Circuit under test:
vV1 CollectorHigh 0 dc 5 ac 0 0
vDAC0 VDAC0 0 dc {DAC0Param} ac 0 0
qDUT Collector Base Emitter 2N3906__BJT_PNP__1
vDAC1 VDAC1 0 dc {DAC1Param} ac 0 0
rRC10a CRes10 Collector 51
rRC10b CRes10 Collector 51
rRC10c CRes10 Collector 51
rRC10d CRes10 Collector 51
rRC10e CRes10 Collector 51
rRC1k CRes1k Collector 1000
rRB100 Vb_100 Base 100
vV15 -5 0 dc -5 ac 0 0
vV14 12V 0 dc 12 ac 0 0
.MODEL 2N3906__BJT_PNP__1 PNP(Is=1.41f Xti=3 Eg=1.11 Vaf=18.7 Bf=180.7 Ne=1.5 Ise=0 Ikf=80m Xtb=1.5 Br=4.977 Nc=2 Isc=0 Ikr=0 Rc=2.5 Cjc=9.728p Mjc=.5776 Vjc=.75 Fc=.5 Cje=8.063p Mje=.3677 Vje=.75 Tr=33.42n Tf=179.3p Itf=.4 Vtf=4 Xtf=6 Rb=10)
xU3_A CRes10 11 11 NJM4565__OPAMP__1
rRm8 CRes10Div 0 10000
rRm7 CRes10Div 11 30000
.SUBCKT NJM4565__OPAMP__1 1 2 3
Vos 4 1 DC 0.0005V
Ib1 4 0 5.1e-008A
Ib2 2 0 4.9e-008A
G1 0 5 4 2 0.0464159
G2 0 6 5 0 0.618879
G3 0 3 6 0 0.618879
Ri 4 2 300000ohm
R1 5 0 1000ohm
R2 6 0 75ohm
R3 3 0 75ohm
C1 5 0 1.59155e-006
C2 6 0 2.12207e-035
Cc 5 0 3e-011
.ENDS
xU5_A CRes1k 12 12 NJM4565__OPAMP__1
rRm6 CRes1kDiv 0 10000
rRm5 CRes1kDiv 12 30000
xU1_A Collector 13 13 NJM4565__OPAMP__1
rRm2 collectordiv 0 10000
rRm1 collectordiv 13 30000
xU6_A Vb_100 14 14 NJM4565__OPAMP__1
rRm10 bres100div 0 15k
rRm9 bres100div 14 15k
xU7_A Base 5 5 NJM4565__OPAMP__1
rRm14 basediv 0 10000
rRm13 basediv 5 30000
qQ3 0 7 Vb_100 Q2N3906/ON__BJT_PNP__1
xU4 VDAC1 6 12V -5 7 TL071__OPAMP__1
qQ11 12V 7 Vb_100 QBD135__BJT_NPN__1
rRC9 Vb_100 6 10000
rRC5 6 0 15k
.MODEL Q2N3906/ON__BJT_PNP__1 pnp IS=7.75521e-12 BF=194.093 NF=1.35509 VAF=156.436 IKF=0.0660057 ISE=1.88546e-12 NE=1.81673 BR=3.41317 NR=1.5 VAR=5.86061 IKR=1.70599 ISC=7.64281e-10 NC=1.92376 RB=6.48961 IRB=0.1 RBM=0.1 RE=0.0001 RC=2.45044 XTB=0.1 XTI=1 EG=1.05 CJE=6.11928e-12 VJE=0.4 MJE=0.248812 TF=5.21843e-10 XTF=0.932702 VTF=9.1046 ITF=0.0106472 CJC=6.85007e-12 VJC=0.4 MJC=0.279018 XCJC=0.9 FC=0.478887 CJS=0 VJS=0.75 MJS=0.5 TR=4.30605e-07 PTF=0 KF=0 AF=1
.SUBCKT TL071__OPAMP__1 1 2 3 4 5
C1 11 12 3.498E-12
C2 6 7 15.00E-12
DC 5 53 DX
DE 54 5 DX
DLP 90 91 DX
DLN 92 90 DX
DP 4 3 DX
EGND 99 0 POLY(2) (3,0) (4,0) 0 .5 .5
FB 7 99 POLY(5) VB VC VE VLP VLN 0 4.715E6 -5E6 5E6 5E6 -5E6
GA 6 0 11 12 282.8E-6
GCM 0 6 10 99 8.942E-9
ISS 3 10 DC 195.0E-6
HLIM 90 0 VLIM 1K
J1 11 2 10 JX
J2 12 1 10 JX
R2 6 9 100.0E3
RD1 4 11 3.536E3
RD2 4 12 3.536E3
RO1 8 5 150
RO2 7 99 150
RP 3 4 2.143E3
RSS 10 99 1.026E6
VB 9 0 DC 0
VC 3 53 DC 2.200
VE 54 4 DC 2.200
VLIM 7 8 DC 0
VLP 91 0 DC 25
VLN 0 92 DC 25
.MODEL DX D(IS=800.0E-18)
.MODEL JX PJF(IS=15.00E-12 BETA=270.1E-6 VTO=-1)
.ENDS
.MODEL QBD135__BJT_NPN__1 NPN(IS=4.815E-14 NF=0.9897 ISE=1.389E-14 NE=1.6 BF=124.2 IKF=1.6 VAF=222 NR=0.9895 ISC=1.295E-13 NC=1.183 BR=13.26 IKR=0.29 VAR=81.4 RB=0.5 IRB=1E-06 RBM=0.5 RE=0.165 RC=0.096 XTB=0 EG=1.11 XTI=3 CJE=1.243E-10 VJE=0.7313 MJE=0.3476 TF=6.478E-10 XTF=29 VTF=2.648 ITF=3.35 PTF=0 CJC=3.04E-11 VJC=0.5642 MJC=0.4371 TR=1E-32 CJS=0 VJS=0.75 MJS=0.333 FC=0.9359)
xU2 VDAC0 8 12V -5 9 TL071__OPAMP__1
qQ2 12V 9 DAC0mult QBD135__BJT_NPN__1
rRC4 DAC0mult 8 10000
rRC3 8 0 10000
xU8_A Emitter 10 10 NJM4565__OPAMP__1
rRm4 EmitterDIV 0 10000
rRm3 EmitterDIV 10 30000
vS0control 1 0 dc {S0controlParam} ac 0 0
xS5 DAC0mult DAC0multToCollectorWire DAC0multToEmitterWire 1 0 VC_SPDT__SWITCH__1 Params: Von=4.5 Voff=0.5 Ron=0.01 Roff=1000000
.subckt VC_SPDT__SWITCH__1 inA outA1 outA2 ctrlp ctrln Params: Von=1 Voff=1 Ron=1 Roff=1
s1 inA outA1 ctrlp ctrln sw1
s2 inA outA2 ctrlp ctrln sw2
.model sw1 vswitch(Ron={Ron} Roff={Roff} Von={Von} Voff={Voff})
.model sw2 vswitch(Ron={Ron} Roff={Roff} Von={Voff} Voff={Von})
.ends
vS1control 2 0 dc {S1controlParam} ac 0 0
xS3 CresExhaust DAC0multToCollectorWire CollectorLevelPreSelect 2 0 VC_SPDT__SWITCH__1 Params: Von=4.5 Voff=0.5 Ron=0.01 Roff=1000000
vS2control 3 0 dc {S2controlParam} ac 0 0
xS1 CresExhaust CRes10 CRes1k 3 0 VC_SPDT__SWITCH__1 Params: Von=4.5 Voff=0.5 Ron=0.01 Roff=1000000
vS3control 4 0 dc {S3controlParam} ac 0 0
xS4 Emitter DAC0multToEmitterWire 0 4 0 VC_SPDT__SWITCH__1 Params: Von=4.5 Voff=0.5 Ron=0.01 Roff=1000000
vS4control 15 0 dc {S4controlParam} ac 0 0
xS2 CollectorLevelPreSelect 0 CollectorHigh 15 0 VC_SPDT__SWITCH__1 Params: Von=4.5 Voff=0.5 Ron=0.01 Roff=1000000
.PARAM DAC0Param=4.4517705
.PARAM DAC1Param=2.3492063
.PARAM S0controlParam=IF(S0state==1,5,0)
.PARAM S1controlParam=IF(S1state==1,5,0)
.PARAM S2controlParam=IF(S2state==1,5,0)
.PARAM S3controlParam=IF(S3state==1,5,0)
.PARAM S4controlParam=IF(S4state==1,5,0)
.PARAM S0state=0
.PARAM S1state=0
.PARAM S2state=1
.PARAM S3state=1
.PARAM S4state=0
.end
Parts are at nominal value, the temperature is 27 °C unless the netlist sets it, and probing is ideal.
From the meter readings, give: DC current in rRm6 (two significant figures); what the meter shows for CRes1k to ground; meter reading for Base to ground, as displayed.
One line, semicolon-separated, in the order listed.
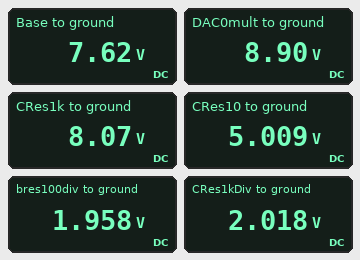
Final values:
200 µA; 8.07 V; 7.62 V
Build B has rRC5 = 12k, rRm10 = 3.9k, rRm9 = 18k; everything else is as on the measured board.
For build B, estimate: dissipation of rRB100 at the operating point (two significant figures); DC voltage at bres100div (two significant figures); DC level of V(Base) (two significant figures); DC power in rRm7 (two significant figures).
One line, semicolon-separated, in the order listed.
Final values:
110 mW; 770 mV; 7.7 V; 470 µW
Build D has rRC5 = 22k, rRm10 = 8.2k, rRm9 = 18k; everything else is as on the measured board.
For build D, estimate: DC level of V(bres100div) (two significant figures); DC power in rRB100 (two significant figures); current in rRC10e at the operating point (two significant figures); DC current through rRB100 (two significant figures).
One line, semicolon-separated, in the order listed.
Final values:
1.1 V; 170 mW; 60 mA; 42 mA
